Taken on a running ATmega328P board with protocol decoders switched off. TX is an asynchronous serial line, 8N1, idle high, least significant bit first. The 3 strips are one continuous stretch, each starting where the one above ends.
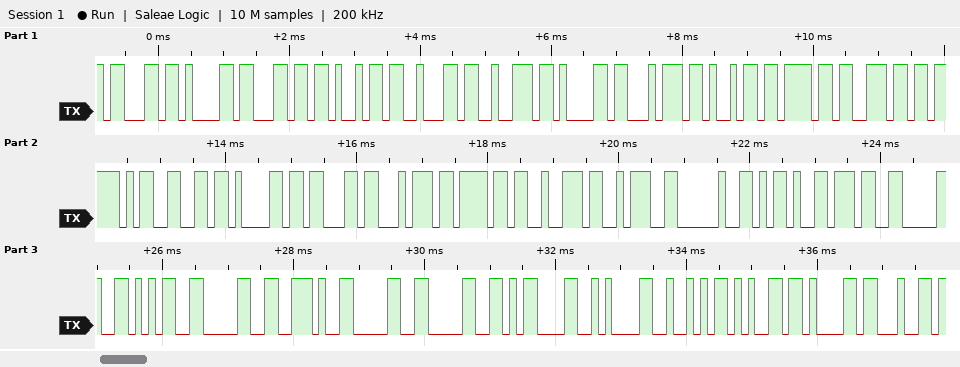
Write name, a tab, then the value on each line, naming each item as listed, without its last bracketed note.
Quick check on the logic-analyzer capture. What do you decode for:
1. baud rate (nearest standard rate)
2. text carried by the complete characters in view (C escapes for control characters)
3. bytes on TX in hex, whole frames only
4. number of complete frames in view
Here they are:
baud rate	9600 baud
text carried by the complete characters in view	"calibration_factor: -7050.00\r\nRead"
bytes on TX in hex, whole frames only	63 61 6C 69 62 72 61 74 69 6F 6E 5F 66 61 63 74 6F 72 3A 20 2D 37 30 35 30 2E 30 30 0D 0A 52 65 61 64
number of complete frames in view	34
